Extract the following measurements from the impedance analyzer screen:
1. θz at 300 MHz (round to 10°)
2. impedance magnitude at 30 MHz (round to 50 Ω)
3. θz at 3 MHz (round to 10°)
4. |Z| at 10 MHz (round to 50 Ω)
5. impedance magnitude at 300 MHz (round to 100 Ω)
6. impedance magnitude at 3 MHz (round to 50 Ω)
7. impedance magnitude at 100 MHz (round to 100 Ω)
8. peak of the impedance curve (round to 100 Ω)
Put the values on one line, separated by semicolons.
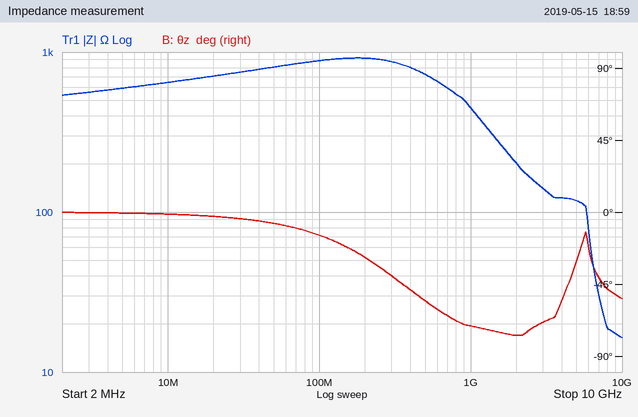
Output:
-40°; 750 Ω; 0°; 650 Ω; 900 Ω; 550 Ω; 900 Ω; 900 Ω
